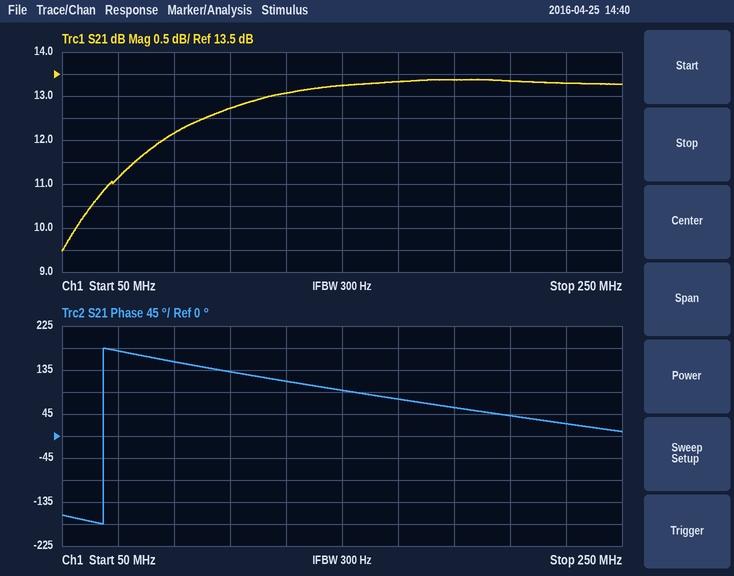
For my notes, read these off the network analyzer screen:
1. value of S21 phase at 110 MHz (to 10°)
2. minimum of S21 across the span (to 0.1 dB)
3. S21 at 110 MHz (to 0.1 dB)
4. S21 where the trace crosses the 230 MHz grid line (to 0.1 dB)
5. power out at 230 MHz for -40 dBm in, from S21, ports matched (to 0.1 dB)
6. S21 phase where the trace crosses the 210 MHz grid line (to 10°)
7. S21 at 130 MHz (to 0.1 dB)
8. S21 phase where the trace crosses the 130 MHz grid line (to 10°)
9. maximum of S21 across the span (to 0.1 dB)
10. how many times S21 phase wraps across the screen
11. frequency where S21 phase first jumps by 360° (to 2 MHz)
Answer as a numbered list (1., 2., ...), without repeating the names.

1. 130°
2. 9.5 dB
3. 12.7 dB
4. 13.3 dB
5. -26.7 dBm
6. 40°
7. 13.1 dB
8. 110°
9. 13.4 dB
10. 1
11. 64 MHz
